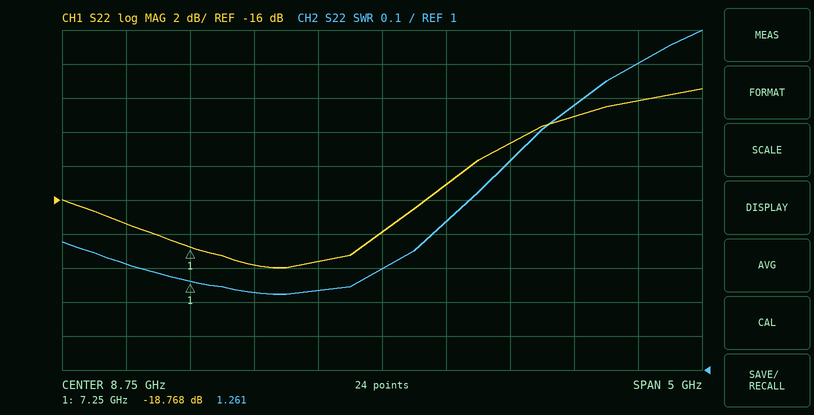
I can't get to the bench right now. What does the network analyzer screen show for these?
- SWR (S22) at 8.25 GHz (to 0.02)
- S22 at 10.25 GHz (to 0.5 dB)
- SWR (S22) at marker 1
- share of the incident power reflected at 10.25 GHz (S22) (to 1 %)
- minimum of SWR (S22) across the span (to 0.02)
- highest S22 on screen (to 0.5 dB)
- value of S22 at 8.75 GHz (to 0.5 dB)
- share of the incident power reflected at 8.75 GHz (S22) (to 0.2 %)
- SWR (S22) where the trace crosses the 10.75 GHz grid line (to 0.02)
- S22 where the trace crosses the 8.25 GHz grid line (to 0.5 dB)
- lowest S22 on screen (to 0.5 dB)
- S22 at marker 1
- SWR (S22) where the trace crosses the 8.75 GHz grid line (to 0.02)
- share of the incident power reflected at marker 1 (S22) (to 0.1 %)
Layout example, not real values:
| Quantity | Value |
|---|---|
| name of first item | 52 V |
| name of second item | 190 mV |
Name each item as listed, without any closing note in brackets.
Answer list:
| Quantity | Value |
|---|---|
| SWR (S22) at 8.25 GHz | 1.24 |
| S22 at 10.25 GHz | -11.0 dB |
| SWR (S22) at marker 1 | 1.261 |
| share of the incident power reflected at 10.25 GHz (S22) | 8 % |
| minimum of SWR (S22) across the span | 1.22 |
| highest S22 on screen | -9.5 dB |
| value of S22 at 8.75 GHz | -18.0 dB |
| share of the incident power reflected at 8.75 GHz (S22) | 1.6 % |
| SWR (S22) where the trace crosses the 10.75 GHz grid line | 1.90 |
| S22 where the trace crosses the 8.25 GHz grid line | -19.5 dB |
| lowest S22 on screen | -20.0 dB |
| S22 at marker 1 | -18.768 dB |
| SWR (S22) where the trace crosses the 8.75 GHz grid line | 1.30 |
| share of the incident power reflected at marker 1 (S22) | 1.3 % |
